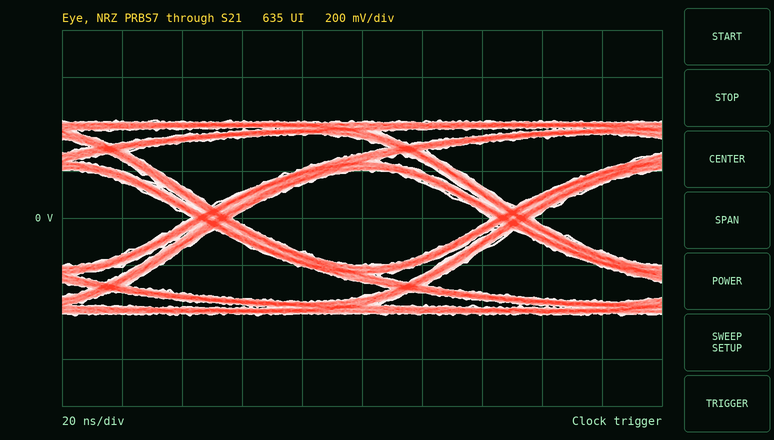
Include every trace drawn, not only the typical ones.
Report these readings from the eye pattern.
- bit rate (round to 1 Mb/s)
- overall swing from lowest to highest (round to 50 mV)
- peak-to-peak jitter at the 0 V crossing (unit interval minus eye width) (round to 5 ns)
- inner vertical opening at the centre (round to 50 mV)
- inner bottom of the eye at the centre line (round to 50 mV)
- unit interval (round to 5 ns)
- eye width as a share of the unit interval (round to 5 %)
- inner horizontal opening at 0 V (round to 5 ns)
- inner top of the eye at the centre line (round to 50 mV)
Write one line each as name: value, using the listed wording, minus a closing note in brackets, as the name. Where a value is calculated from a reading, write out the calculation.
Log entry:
bit rate: 10 Mb/s
overall swing from lowest to highest: 850 mV
peak-to-peak jitter at the 0 V crossing (unit interval minus eye width): 15 ns
inner vertical opening at the centre: 400 mV
inner bottom of the eye at the centre line: -200 mV
unit interval: 100 ns
eye width as a share of the unit interval: 85 ns / 100 ns ≈ 85 %
inner horizontal opening at 0 V: 85 ns
inner top of the eye at the centre line: 200 mV
